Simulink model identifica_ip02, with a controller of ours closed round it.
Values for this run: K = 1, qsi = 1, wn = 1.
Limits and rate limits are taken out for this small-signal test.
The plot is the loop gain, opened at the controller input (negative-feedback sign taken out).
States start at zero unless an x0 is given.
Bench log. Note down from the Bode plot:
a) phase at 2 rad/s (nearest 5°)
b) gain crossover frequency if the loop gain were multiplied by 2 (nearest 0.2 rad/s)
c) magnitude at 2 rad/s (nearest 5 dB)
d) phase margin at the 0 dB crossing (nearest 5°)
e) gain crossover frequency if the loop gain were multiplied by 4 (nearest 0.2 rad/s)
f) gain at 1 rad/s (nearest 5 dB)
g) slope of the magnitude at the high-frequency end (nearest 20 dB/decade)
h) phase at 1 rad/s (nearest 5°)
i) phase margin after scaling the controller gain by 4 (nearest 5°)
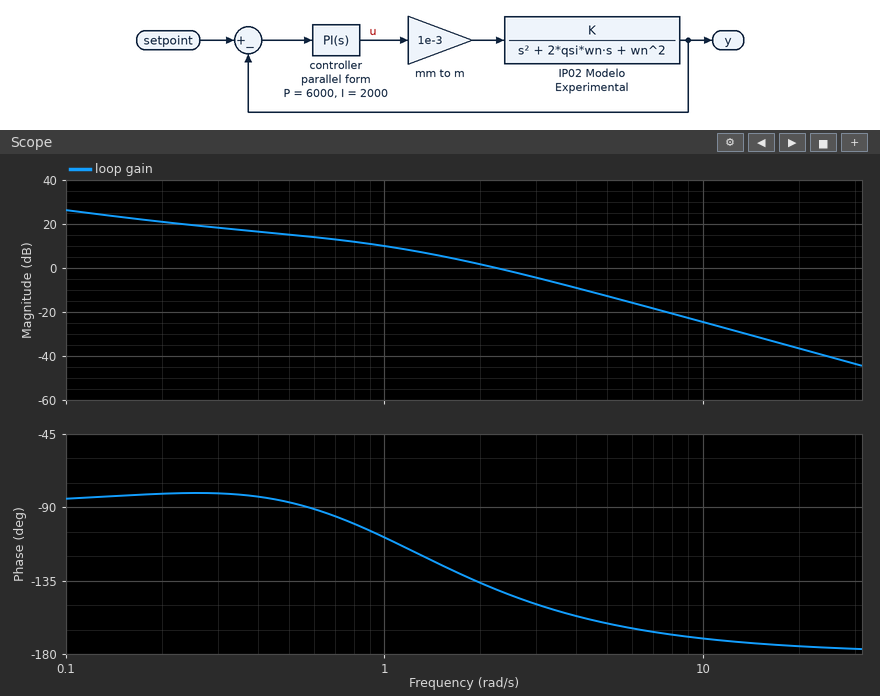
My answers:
-135°
3.4 rad/s
0 dB
40°
4.8 rad/s
10 dB
-40 dB/decade
-110°
20°
